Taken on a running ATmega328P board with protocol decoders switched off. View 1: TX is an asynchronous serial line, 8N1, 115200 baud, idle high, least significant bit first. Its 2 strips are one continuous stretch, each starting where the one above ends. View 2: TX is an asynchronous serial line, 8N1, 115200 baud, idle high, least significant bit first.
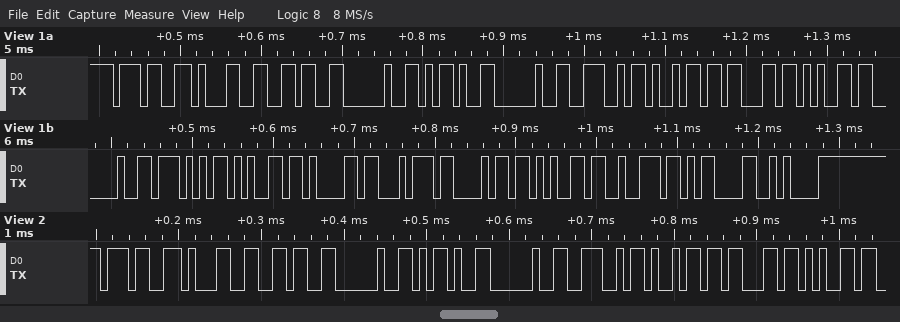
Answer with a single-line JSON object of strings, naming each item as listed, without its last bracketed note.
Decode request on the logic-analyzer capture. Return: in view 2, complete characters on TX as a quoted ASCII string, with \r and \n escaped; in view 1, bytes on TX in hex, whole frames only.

{"in view 2, complete characters on TX as a quoted ASCII string, with \\r and \\n escaped": "\"716 - Nice\"", "in view 1, bytes on TX in hex, whole frames only": "0x37 0x31 0x36 0x20 0x2D 0x20 0x4E 0x69 0x63 0x65 0x20 0x57 0x65 0x61 0x74 0x68 0x65 0x72 0x0D 0x0A"}
